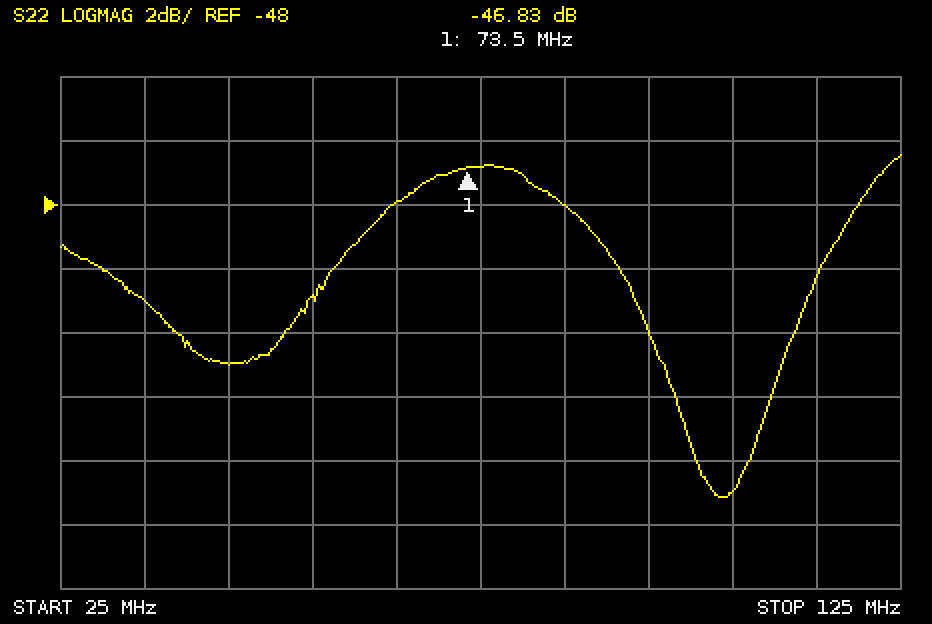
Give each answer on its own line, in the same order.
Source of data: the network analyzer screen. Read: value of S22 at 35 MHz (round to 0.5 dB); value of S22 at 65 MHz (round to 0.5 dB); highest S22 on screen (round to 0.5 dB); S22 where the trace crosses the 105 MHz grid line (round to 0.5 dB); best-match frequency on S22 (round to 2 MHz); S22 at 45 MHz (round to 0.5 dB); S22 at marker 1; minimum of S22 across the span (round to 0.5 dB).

-51.0 dB
-48.0 dB
-46.5 dB
-57.0 dB
104 MHz
-53.0 dB
-46.83 dB
-57.0 dB
